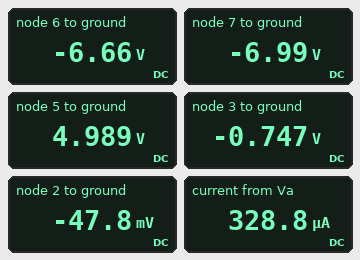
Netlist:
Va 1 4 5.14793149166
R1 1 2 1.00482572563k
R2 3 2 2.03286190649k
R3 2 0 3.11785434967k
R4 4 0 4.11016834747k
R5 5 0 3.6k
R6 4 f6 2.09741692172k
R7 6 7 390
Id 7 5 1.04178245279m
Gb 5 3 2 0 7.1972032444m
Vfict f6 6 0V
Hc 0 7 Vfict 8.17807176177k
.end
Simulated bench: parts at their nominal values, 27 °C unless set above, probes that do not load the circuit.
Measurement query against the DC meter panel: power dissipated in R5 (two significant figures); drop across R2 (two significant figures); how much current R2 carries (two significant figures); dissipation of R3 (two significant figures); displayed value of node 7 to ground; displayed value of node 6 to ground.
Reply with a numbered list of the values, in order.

1. 6.9 mW
2. 700 mV
3. 340 µA
4. 730 nW
5. -6.99 V
6. -6.66 V
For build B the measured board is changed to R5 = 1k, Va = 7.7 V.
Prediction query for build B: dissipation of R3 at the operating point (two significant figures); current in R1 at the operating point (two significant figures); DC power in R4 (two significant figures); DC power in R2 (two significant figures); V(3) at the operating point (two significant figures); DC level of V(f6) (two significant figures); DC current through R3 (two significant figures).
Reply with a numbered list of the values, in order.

1. 1.6 µW
2. 490 µA
3. 13 mW
4. 540 µW
5. -1.1 V
6. -10 V
7. 23 µA
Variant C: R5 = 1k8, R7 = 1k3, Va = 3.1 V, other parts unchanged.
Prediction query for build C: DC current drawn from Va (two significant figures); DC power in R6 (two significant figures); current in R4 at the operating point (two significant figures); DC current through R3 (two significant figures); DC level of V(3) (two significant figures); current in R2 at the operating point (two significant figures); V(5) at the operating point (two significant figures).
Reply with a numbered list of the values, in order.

1. 100 µA
2. 830 µW
3. 730 µA
4. 4.8 µA
5. -230 mV
6. 110 µA
7. 2.1 V
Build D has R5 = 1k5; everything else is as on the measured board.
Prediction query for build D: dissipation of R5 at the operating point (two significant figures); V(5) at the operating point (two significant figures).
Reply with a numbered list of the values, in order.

1. 2.9 mW
2. 2.1 V
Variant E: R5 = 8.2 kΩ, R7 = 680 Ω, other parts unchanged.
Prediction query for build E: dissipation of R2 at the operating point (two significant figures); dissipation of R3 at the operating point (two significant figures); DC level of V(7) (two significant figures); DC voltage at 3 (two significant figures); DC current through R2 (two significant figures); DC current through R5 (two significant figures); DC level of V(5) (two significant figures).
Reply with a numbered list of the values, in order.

1. 180 µW
2. 550 nW
3. -7.4 V
4. -650 mV
5. 300 µA
6. 1.3 mA
7. 11 V
